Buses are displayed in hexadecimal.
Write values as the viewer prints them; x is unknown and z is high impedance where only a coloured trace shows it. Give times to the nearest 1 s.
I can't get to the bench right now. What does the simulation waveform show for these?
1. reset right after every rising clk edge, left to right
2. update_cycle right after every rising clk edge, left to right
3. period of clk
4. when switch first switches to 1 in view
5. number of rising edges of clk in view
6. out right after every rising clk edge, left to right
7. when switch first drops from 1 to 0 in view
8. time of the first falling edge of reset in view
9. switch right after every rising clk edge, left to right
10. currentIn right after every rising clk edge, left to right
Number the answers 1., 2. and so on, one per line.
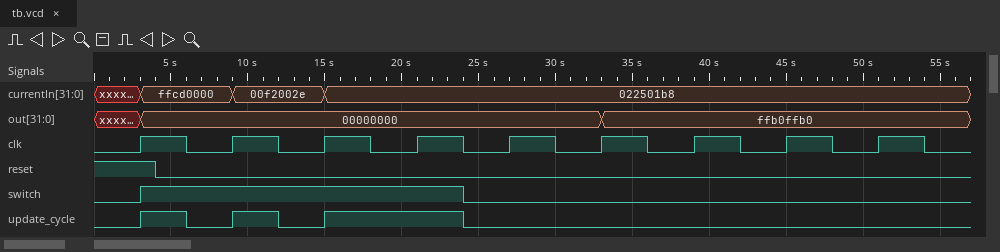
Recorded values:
1. 1 0 0 0 0 0 0 0 0
2. 1 1 1 1 0 0 0 0 0
3. 6 s
4. 3 s
5. 9
6. 00000000, 00000000, 00000000, 00000000, 00000000, ffb0ffb0, ffb0ffb0, ffb0ffb0, ffb0ffb0
7. 24 s
8. 4 s
9. 1 1 1 1 0 0 0 0 0
10. ffcd0000, 00f2002e, 022501b8, 022501b8, 022501b8, 022501b8, 022501b8, 022501b8, 022501b8
